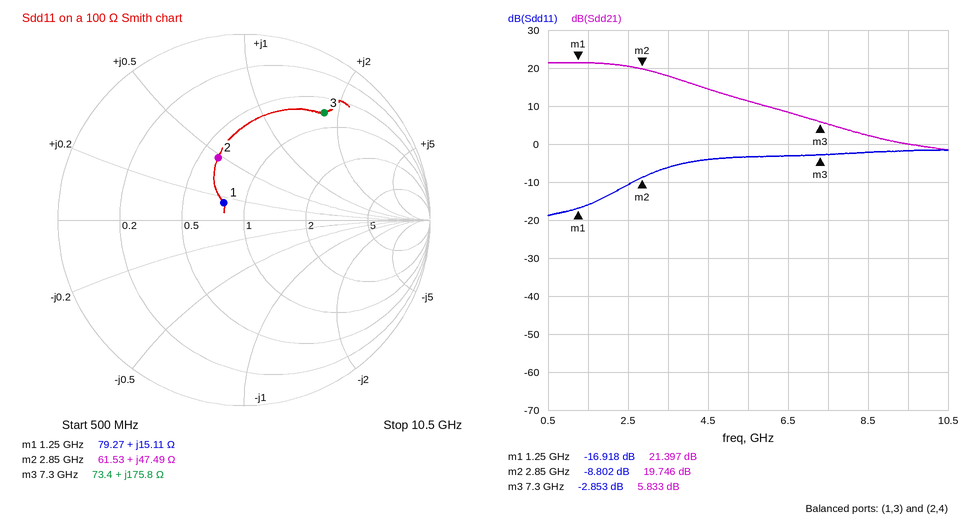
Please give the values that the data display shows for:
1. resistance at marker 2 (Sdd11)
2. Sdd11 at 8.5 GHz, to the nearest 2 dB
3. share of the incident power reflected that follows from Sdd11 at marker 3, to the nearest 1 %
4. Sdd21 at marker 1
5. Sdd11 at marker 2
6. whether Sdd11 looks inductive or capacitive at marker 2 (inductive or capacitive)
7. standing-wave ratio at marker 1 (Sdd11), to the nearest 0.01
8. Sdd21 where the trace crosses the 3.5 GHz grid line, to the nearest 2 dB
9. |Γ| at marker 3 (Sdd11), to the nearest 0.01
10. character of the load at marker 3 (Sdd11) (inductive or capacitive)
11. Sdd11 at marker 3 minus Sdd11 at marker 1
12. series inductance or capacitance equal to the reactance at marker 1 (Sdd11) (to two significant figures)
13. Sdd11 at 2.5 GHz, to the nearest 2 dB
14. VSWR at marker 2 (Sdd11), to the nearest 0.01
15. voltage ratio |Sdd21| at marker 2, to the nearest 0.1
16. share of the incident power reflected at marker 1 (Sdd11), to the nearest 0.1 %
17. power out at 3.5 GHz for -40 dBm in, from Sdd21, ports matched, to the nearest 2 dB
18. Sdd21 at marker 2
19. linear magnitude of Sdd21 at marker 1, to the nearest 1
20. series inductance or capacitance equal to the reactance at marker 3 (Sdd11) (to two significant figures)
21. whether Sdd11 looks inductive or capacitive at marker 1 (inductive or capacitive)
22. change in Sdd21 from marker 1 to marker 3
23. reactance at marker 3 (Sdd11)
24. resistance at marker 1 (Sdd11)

61.53 Ω
-2 dB
52 %
21.397 dB
-8.802 dB
inductive
1.33
18 dB
0.72
inductive
14.065 dB
1.9 nH
-10 dB
2.14
9.7
2.0 %
-22 dBm
19.746 dB
12
3.8 nH
inductive
-15.564 dB
+175.8 Ω
79.27 Ω
